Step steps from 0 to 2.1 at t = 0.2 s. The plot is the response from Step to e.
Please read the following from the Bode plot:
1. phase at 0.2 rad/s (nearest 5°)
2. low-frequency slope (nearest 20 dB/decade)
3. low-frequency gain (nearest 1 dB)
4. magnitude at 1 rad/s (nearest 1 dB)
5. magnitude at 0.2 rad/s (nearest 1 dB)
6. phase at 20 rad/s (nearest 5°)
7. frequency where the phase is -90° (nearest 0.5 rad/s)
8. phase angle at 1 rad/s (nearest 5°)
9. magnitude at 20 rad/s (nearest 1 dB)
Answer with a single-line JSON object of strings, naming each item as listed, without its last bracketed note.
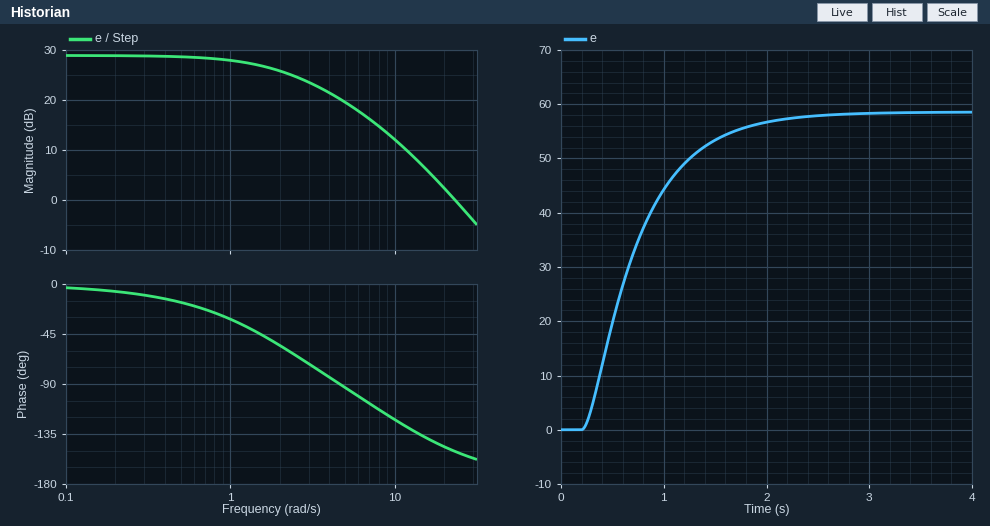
{"phase at 0.2 rad/s": "-5°", "low-frequency slope": "0 dB/decade", "low-frequency gain": "29 dB", "magnitude at 1 rad/s": "28 dB", "magnitude at 0.2 rad/s": "29 dB", "phase at 20 rad/s": "-145°", "frequency where the phase is -90°": "4.5 rad/s", "phase angle at 1 rad/s": "-30°", "magnitude at 20 rad/s": "2 dB"}
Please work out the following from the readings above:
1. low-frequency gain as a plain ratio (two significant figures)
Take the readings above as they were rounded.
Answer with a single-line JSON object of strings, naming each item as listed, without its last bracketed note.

{"low-frequency gain as a plain ratio": "28"}
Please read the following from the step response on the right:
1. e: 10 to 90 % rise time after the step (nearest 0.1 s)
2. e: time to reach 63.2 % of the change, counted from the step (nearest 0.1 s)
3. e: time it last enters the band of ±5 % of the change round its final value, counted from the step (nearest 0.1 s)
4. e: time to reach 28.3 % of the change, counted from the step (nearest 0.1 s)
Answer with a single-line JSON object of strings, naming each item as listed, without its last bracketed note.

{"e: 10 to 90 % rise time after the step": "1.1 s", "e: time to reach 63.2 % of the change, counted from the step": "0.6 s", "e: time it last enters the band of ±5 % of the change round its final value, counted from the step": "1.6 s", "e: time to reach 28.3 % of the change, counted from the step": "0.3 s"}
